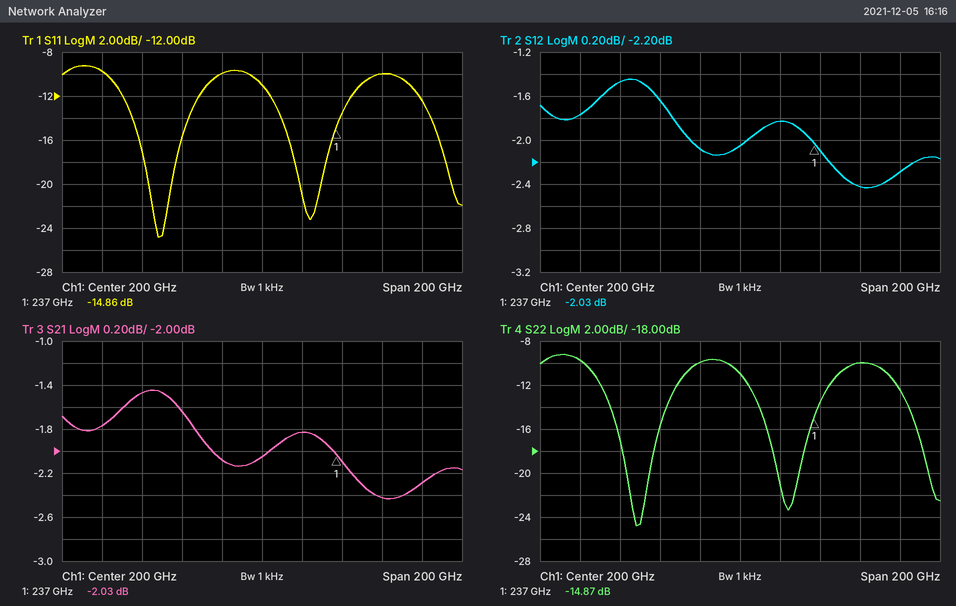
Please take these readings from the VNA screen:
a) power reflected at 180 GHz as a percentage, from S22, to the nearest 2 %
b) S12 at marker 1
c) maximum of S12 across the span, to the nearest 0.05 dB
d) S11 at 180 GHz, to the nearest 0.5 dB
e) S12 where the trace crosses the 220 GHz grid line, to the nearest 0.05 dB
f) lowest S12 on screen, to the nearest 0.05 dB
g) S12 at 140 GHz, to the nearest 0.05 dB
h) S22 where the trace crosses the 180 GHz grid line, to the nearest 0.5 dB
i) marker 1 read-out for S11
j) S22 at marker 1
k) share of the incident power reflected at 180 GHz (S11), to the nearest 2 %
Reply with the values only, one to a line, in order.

10 %
-2.03 dB
-1.45 dB
-10.0 dB
-1.85 dB
-2.45 dB
-1.45 dB
-10.0 dB
-14.86 dB
-14.87 dB
10 %
